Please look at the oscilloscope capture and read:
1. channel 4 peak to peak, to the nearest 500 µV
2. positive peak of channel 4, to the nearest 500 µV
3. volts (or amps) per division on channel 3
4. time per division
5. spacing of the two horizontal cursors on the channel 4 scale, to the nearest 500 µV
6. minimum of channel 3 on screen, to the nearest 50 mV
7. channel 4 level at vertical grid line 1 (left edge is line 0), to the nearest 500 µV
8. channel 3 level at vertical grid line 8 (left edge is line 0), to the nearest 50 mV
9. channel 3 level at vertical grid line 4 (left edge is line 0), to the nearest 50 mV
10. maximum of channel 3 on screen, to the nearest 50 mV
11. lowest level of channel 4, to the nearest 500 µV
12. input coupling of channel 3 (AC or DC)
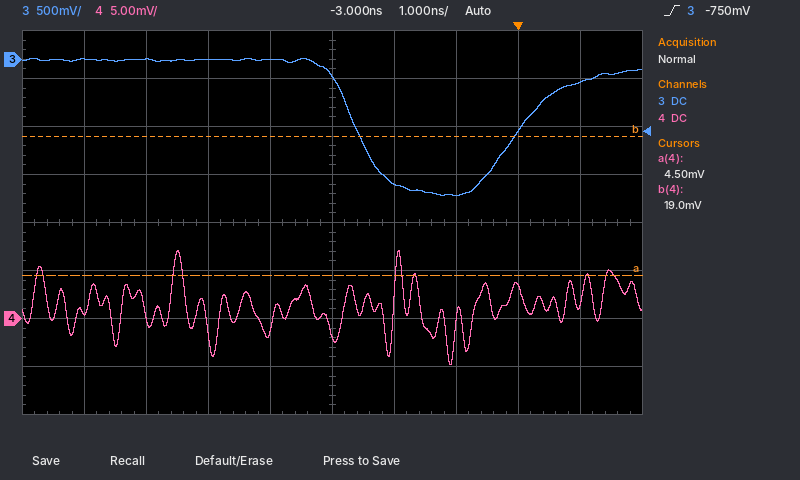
12.0 mV
7.0 mV
500 mV
1 ns
14.5 mV
-1.40 V
500 µV
-750 mV
0 mV
0 mV
-5.0 mV
DC
